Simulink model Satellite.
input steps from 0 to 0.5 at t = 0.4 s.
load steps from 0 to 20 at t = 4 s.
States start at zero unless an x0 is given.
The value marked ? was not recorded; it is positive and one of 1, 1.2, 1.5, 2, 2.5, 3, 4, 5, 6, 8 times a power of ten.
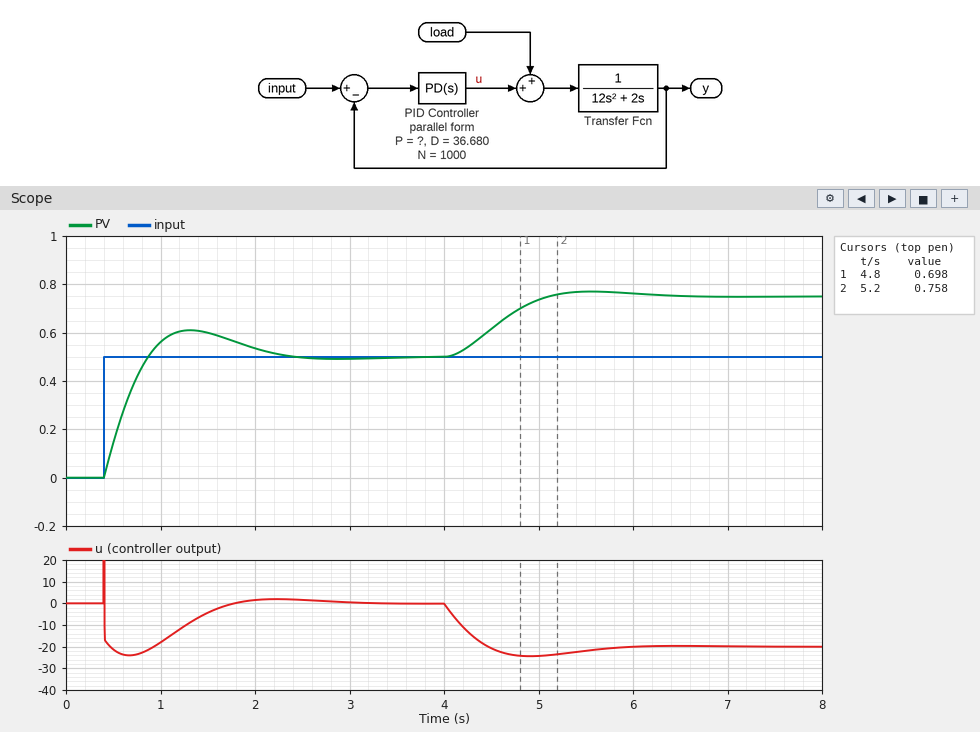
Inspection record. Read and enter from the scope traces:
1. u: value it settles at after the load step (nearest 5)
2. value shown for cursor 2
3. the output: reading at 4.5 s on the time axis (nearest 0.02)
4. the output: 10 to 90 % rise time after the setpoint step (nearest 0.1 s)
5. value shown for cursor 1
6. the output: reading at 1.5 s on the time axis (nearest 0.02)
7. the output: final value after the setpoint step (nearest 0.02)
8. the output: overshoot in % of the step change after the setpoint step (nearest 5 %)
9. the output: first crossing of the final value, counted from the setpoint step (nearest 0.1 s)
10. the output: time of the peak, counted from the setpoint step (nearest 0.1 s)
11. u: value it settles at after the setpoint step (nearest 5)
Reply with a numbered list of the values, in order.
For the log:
1. -20
2. 0.758
3. 0.62
4. 0.4 s
5. 0.698
6. 0.60
7. 0.50
8. 20 %
9. 0.5 s
10. 0.9 s
11. 0
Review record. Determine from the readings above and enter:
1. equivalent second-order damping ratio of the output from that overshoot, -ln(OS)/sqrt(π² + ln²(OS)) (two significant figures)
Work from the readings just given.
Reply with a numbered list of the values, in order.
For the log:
1. 0.46
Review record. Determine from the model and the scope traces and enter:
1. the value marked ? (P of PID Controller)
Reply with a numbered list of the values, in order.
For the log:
1. 80
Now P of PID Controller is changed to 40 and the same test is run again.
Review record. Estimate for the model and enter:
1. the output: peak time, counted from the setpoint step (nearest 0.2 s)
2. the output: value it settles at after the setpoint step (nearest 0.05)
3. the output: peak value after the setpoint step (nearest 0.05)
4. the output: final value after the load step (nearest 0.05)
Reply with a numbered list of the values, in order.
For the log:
1. 1.2 s
2. 0.50
3. 0.55
4. 1.00
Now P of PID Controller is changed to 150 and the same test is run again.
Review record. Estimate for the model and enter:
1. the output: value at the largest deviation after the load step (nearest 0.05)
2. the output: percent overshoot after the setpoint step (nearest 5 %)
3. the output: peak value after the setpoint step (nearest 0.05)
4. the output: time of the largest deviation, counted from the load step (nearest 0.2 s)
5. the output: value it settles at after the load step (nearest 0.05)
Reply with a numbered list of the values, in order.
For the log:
1. 0.65
2. 30 %
3. 0.65
4. 1.0 s
5. 0.65
